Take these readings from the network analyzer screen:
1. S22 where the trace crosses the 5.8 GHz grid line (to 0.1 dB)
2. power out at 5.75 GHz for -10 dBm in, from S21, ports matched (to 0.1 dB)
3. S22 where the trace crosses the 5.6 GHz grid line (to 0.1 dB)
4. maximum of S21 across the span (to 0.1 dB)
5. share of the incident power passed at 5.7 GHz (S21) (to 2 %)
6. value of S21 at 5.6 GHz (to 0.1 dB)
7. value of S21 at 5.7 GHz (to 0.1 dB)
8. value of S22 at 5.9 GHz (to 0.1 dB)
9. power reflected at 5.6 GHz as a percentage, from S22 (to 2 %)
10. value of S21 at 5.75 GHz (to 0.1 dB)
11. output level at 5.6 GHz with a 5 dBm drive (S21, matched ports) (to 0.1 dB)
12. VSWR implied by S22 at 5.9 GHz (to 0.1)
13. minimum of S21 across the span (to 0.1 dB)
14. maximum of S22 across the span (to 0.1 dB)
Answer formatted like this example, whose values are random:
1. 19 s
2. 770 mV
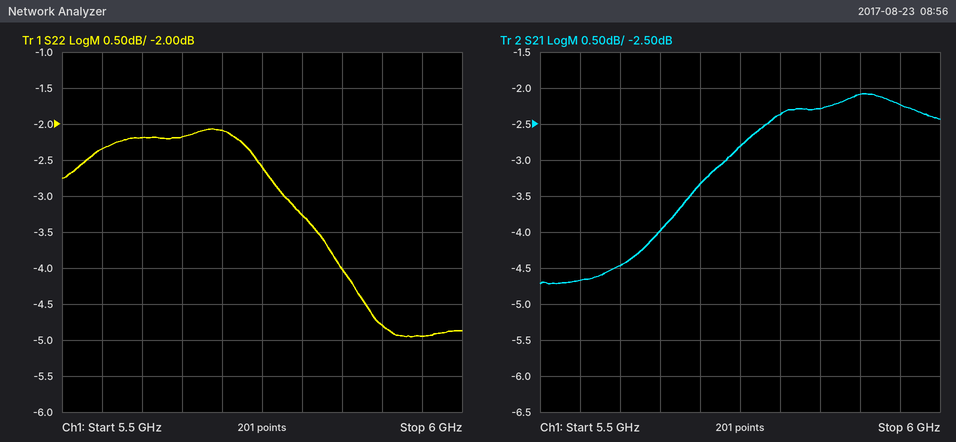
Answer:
1. -3.3 dB
2. -12.8 dBm
3. -2.2 dB
4. -2.1 dB
5. 46 %
6. -4.5 dB
7. -3.3 dB
8. -4.8 dB
9. 60 %
10. -2.8 dB
11. 0.5 dBm
12. 3.7
13. -4.7 dB
14. -2.1 dB
